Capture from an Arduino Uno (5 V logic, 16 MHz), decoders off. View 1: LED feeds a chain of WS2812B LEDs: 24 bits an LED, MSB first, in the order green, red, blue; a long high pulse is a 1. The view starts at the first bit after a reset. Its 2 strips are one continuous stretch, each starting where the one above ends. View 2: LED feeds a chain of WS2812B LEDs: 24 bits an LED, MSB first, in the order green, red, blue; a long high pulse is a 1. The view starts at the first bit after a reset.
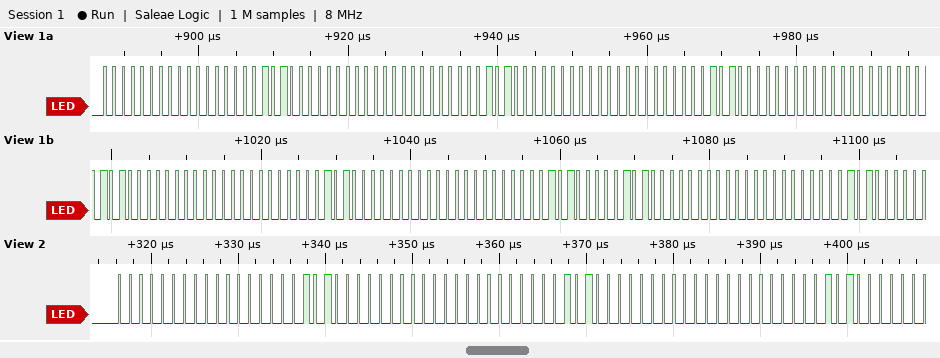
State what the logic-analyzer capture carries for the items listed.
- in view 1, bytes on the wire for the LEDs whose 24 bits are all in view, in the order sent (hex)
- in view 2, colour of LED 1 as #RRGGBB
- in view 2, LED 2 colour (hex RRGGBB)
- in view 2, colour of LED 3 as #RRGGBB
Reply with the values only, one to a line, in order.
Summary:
00 00 50 00 00 50 00 00 50 00 00 50 00 00 50 00 00 50 50 00 00
#000050
#000050
#000050
